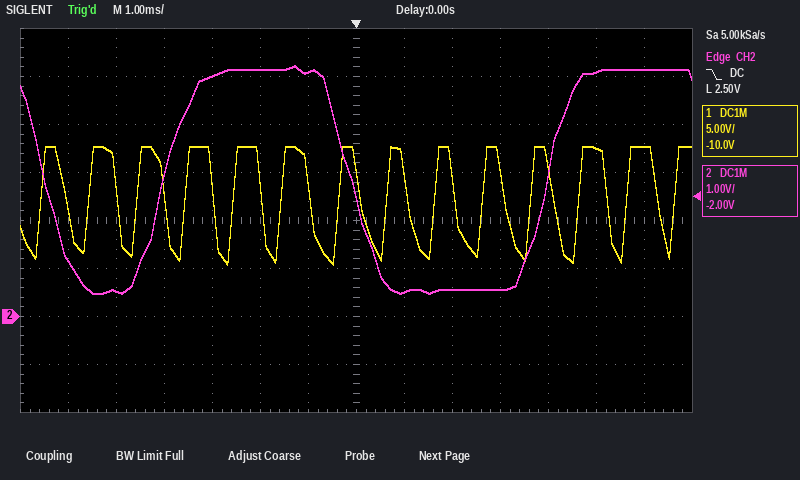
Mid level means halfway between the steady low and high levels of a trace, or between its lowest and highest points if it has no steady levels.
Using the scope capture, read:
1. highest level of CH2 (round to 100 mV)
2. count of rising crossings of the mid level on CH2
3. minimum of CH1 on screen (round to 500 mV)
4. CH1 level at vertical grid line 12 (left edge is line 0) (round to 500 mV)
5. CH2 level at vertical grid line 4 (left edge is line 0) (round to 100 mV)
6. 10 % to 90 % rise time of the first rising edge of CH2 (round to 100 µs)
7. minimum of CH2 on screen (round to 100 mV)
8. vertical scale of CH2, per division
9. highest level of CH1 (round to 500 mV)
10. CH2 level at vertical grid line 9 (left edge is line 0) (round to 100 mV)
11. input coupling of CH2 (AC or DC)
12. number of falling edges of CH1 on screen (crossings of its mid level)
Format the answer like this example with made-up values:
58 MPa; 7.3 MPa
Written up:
5.2 V; 2; 5.5 V; 17.5 V; 5.0 V; 1.2 ms; 500 mV; 1 V; 17.5 V; 600 mV; DC; 13
